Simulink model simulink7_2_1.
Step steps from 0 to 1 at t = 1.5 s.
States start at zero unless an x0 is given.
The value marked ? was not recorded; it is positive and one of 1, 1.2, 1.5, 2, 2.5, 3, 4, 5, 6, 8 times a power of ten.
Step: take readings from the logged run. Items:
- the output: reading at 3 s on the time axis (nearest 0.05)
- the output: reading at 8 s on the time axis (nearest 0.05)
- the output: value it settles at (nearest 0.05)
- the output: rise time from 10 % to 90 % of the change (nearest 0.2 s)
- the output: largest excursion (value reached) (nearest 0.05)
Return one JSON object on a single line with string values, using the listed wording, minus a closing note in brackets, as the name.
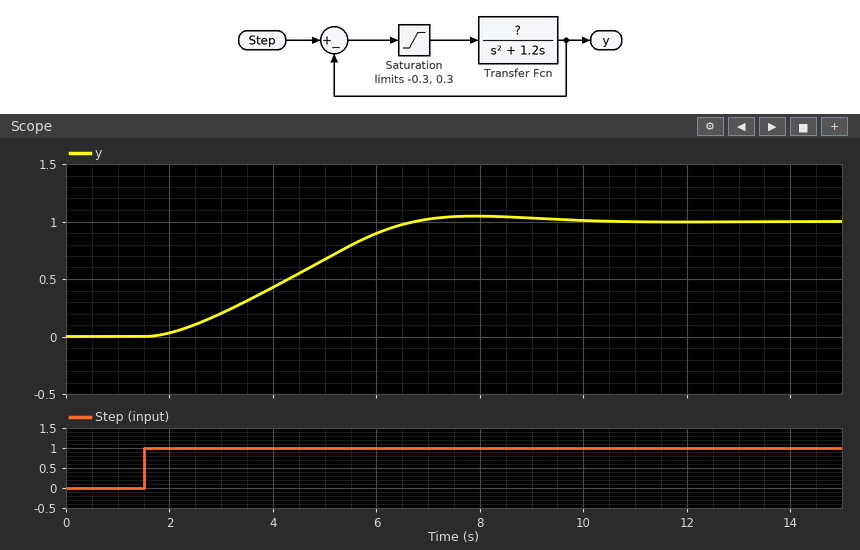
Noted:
{"the output: reading at 3 s on the time axis": "0.20", "the output: reading at 8 s on the time axis": "1.05", "the output: value it settles at": "1.00", "the output: rise time from 10 % to 90 % of the change": "3.6 s", "the output: largest excursion (value reached)": "1.05"}
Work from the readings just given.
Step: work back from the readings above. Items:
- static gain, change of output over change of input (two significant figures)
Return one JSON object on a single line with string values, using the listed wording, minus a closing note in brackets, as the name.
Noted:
{"static gain, change of output over change of input": "1.0"}
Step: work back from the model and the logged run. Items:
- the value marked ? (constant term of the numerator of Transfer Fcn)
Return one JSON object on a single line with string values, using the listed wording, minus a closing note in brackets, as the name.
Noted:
{"the value marked ?": "1"}
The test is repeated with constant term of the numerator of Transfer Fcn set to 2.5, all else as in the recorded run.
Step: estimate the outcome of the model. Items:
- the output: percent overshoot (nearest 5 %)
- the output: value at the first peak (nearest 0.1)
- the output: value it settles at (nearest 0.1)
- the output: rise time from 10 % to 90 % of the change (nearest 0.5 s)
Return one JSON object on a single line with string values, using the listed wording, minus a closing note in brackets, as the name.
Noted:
{"the output: percent overshoot": "15 %", "the output: value at the first peak": "1.2", "the output: value it settles at": "1.0", "the output: rise time from 10 % to 90 % of the change": "1.5 s"}
